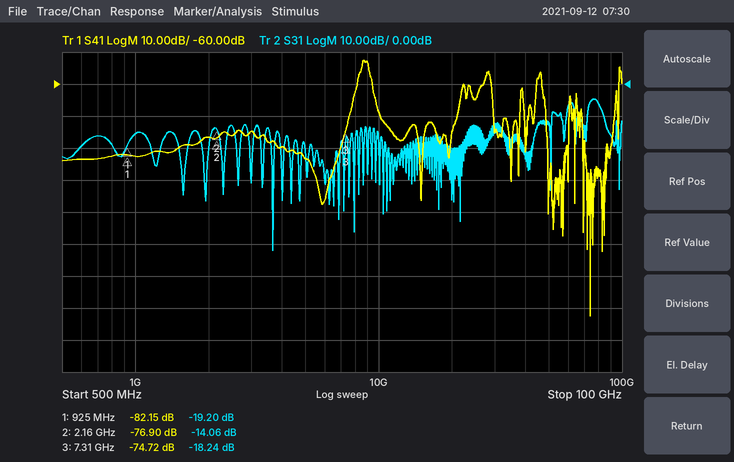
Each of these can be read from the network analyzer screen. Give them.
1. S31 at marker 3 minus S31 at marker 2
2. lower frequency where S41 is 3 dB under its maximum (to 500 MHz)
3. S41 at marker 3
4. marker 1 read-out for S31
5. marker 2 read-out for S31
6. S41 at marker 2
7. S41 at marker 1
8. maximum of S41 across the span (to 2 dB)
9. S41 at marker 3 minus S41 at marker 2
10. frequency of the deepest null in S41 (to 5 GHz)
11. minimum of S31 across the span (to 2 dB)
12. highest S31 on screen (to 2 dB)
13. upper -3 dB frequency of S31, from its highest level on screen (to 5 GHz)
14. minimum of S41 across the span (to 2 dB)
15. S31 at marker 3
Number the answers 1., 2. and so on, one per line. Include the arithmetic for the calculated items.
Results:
1. -18.24 − (-14.06) = -4.18 dB
2. 8.5 GHz
3. -74.72 dB
4. -19.20 dB
5. -14.06 dB
6. -76.90 dB
7. -82.15 dB
8. -52 dB
9. -74.72 − (-76.9) = 2.18 dB
10. 75 GHz
11. -52 dB
12. -4 dB
13. 80 GHz
14. -132 dB
15. -18.24 dB
